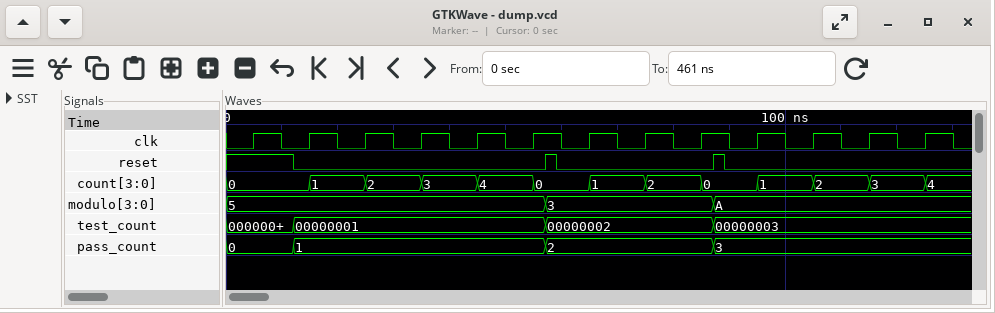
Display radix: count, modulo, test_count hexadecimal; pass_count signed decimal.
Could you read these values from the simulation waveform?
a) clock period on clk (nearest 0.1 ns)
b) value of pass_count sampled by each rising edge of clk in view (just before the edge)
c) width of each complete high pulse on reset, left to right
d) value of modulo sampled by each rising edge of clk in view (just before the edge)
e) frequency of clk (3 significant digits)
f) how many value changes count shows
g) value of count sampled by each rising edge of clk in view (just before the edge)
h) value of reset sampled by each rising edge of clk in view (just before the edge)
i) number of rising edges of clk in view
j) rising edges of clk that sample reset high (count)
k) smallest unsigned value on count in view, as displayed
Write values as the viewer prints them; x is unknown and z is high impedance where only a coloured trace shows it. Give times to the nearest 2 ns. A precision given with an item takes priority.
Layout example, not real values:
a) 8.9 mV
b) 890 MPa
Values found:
a) 10 ns
b) 0, 1, 1, 1, 1, 1, 2, 2, 2, 3, 3, 3, 3
c) 2 ns, 2 ns
d) 5, 5, 5, 5, 5, 5, 3, 3, 3, A, A, A, A
e) 100 MHz
f) 12
g) 0, 0, 1, 2, 3, 4, 0, 1, 2, 0, 1, 2, 3
h) 1 0 0 0 0 0 0 0 0 0 0 0 0
i) 13
j) 1
k) 0
